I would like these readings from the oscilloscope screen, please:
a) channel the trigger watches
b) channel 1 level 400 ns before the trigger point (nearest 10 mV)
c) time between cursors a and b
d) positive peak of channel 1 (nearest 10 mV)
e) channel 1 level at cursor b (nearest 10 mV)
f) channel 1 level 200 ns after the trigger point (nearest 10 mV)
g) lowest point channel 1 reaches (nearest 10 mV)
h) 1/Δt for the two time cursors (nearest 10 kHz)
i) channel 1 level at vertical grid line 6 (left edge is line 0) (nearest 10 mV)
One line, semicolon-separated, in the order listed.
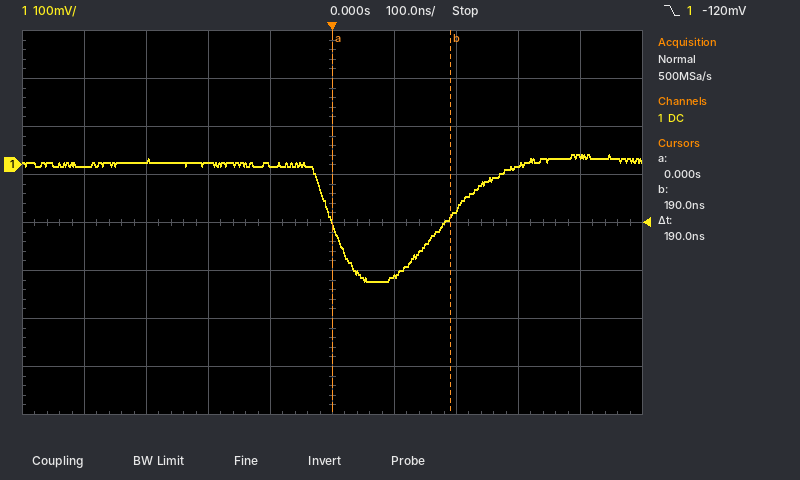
channel 1; 0 mV; 190 ns; 20 mV; -110 mV; -90 mV; -240 mV; 5.26 MHz; -230 mV
